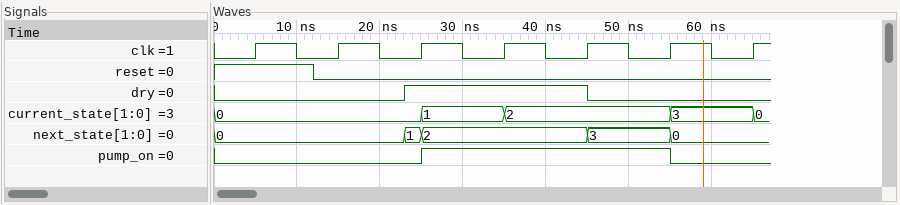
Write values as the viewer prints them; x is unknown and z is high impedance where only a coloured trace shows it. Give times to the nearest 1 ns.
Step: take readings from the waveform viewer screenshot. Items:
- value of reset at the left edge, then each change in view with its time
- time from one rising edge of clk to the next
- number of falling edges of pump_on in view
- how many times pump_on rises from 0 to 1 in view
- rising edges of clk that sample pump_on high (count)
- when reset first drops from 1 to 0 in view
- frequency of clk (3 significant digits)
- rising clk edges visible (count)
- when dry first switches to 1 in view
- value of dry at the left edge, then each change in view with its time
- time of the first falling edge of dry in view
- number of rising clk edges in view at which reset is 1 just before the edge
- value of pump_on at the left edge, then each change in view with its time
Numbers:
1, 0 at 12 ns
10 ns
1
1
3
12 ns
100 MHz
7
23 ns
0, 1 at 23 ns, 0 at 45 ns
45 ns
1
0, 1 at 25 ns, 0 at 55 ns
